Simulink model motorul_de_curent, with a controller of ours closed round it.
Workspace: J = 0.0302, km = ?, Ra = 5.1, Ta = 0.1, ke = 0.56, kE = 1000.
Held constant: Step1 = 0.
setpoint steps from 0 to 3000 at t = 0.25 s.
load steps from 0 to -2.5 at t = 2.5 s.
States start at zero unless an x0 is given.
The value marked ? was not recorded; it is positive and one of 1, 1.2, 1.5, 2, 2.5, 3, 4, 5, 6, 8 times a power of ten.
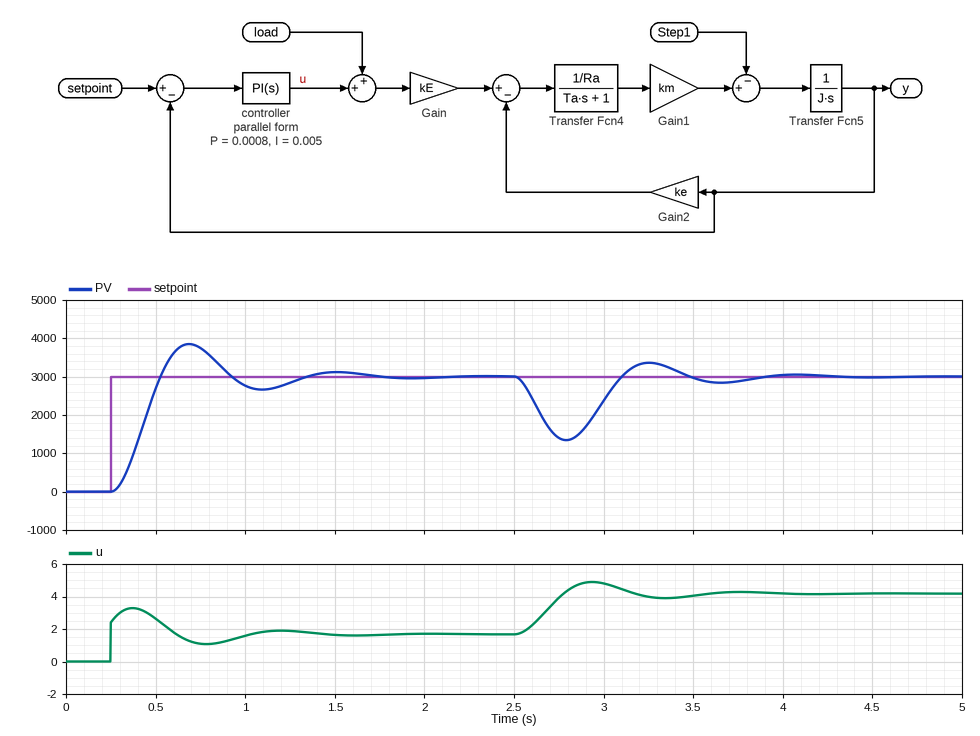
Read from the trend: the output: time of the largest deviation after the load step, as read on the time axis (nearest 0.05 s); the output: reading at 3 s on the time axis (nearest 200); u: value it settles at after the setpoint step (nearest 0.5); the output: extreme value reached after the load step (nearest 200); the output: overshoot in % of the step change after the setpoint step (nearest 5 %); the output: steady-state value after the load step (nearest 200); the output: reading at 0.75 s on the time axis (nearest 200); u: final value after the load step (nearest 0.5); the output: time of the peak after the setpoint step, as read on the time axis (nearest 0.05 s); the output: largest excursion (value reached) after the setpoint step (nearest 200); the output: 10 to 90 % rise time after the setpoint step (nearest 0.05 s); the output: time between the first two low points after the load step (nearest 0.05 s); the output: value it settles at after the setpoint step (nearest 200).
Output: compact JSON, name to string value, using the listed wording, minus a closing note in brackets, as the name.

{"the output: time of the largest deviation after the load step, as read on the time axis": "2.80 s", "the output: reading at 3 s on the time axis": "2400", "u: value it settles at after the setpoint step": "1.5", "the output: extreme value reached after the load step": "1400", "the output: overshoot in % of the step change after the setpoint step": "30 %", "the output: steady-state value after the load step": "3000", "the output: reading at 0.75 s on the time axis": "3800", "u: final value after the load step": "4.0", "the output: time of the peak after the setpoint step, as read on the time axis": "0.70 s", "the output: largest excursion (value reached) after the setpoint step": "3800", "the output: 10 to 90 % rise time after the setpoint step": "0.20 s", "the output: time between the first two low points after the load step": "0.85 s", "the output: value it settles at after the setpoint step": "3000"}
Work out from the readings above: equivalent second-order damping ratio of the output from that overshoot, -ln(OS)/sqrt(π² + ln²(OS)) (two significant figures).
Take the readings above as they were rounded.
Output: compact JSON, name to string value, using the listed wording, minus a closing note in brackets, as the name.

{"equivalent second-order damping ratio of the output from that overshoot, -ln(OS)/sqrt(π² + ln²(OS))": "0.36"}
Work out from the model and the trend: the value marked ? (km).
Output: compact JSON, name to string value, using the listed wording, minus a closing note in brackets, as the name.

{"the value marked ?": "1"}
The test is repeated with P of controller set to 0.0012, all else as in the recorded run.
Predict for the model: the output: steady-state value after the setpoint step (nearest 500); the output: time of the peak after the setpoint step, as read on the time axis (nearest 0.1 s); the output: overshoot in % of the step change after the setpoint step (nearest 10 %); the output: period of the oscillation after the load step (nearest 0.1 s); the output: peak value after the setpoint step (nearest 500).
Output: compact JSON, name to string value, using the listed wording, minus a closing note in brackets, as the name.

{"the output: steady-state value after the setpoint step": "3000", "the output: time of the peak after the setpoint step, as read on the time axis": "0.6 s", "the output: overshoot in % of the step change after the setpoint step": "20 %", "the output: period of the oscillation after the load step": "0.7 s", "the output: peak value after the setpoint step": "3500"}
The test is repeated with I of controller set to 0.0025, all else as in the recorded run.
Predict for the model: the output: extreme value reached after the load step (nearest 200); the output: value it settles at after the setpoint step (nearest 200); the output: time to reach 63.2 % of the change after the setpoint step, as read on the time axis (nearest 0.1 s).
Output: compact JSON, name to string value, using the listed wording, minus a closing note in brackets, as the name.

{"the output: extreme value reached after the load step": "1200", "the output: value it settles at after the setpoint step": "3000", "the output: time to reach 63.2 % of the change after the setpoint step, as read on the time axis": "0.5 s"}
